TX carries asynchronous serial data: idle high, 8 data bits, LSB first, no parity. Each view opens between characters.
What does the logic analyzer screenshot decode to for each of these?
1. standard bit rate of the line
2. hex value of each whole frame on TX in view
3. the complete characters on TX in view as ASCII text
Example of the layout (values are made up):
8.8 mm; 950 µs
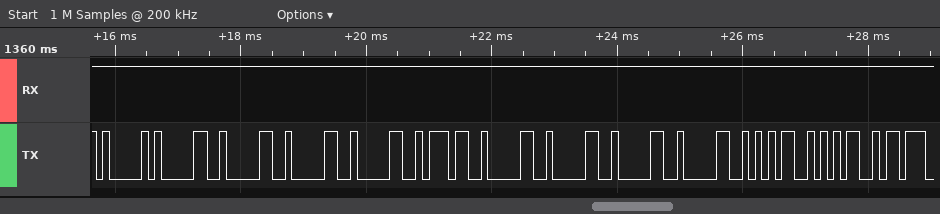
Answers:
9600 baud; 41, 30, 30, 30, 30, 37, 30, 30, 30, 30, 35, 35; "A00007000055"
